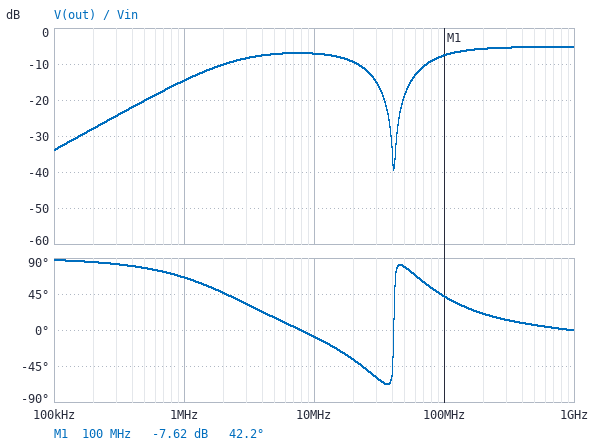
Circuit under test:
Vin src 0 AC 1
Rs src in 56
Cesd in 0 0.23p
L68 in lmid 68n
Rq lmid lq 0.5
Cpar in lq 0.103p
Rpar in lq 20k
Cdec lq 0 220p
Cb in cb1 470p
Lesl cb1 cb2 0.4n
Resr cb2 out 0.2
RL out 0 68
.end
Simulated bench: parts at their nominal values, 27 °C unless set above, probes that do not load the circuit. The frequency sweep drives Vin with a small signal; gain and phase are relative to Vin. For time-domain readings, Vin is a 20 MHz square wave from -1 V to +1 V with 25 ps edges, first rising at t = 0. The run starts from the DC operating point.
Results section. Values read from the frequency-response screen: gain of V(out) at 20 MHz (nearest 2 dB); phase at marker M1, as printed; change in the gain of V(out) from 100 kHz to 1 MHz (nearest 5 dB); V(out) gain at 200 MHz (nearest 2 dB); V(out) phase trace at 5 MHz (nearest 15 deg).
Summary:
-10 dB
42.2 deg
20 dB
-6 dB
15 deg
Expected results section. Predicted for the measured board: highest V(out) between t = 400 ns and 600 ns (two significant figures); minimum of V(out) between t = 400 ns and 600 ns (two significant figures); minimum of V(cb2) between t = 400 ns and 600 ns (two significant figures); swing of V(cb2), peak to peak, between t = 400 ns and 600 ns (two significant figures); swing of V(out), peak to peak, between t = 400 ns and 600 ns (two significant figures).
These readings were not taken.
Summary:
640 mV
-640 mV
-640 mV
1.3 V
1.3 V
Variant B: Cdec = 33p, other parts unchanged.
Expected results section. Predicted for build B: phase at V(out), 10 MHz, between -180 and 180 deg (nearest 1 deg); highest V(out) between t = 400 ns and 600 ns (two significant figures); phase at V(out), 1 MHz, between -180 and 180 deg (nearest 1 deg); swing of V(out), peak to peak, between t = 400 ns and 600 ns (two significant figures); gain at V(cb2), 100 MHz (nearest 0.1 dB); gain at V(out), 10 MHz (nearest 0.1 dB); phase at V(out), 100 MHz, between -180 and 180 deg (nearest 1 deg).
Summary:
11 deg
740 mV
69 deg
1.5 V
-20.6 dB
-5.7 dB
-71 deg
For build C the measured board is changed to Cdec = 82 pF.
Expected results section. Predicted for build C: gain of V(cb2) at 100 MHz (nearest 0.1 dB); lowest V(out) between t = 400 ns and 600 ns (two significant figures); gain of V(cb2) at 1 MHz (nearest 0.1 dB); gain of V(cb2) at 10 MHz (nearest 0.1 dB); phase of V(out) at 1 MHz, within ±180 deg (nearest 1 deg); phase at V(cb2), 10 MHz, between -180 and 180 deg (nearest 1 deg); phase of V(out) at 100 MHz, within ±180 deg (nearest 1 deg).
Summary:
-9.6 dB
-650 mV
-14.5 dB
-5.9 dB
68 deg
6 deg
54 deg
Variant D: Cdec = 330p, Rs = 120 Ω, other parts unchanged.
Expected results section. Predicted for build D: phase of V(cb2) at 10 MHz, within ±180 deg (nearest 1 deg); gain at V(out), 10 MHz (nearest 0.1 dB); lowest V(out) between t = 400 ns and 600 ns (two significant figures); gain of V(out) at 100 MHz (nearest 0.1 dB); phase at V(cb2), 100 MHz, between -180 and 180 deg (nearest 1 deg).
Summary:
-28 deg
-13.5 dB
-500 mV
-12.4 dB
50 deg
